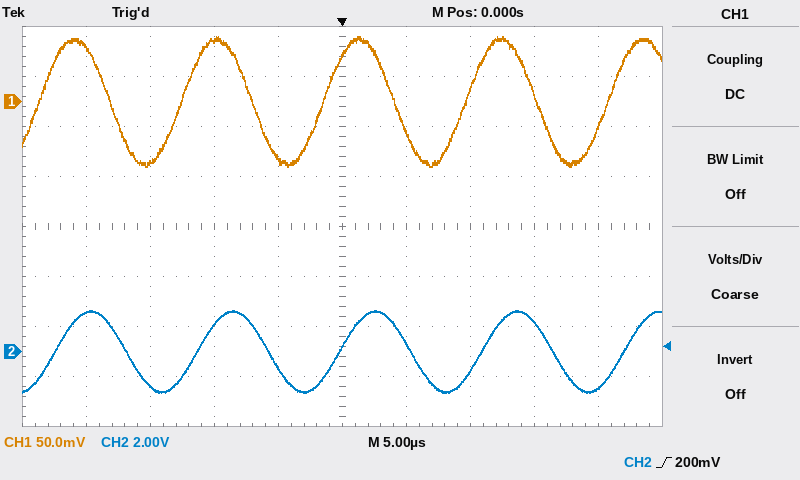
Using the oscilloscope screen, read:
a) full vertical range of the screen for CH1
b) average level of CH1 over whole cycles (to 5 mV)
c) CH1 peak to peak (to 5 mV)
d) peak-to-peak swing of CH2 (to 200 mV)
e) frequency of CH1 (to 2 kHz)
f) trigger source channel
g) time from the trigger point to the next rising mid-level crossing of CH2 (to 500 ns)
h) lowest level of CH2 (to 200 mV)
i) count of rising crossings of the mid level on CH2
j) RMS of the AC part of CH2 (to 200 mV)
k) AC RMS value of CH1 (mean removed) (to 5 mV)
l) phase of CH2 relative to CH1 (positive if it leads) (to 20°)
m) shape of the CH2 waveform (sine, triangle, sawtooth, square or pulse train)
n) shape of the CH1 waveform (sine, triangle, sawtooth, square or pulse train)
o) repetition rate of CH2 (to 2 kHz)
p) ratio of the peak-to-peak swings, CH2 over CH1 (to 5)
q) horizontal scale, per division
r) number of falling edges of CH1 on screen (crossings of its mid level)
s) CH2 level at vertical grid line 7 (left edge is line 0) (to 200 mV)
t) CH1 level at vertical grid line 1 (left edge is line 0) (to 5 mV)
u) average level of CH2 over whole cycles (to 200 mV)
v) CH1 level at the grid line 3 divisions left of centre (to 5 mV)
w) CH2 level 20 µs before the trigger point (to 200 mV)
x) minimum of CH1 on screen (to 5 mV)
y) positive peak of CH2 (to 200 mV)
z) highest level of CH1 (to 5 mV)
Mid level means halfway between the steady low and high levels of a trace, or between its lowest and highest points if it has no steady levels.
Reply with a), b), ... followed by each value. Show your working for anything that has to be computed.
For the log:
a) 400 mV
b) (65 mV + (-65 mV)) / 2 ≈ 0 mV
c) 65 mV − (-65 mV) = 130 mV
d) 1.6 V − (-1.6 V) = 3.2 V
e) 90 kHz
f) CH2
g) 11.0 µs
h) -1.6 V
i) 5
j) 3.2 V / (2√2) ≈ 1.13 V, so 1.2 V to the nearest 200 mV
k) 130 mV / (2√2) ≈ 46.0 mV, so 45 mV to the nearest 5 mV
l) -40°
m) sine
n) sine
o) 90 kHz
p) 3.2 V / 130 mV ≈ 25
q) 5 µs
r) 4
s) -800 mV
t) 55 mV
u) (1.6 V + (-1.6 V)) / 2 ≈ 0.0 V
v) -60 mV
w) 1.6 V
x) -65 mV
y) 1.6 V
z) 65 mV
